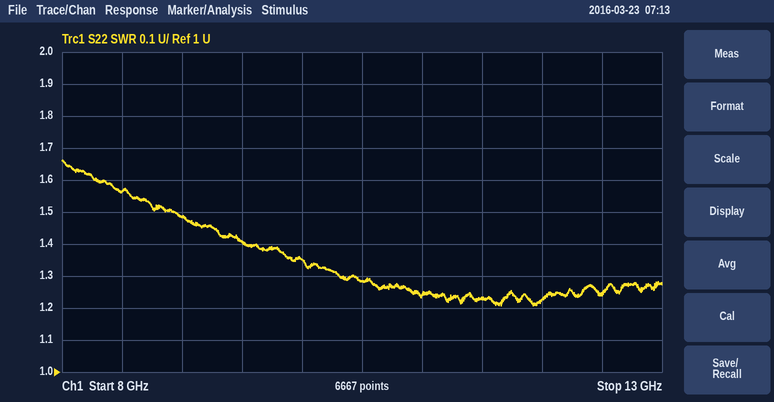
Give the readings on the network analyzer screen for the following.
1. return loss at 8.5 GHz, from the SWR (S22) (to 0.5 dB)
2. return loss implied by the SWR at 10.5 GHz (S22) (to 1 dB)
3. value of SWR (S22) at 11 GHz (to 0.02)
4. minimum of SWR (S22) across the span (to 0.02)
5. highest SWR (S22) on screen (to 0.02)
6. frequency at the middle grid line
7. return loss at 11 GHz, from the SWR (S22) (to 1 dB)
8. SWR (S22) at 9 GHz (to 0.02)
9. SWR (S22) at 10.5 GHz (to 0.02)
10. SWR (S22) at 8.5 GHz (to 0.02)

13.0 dB
18 dB
1.24
1.20
1.66
10.5 GHz
19 dB
1.48
1.28
1.56
